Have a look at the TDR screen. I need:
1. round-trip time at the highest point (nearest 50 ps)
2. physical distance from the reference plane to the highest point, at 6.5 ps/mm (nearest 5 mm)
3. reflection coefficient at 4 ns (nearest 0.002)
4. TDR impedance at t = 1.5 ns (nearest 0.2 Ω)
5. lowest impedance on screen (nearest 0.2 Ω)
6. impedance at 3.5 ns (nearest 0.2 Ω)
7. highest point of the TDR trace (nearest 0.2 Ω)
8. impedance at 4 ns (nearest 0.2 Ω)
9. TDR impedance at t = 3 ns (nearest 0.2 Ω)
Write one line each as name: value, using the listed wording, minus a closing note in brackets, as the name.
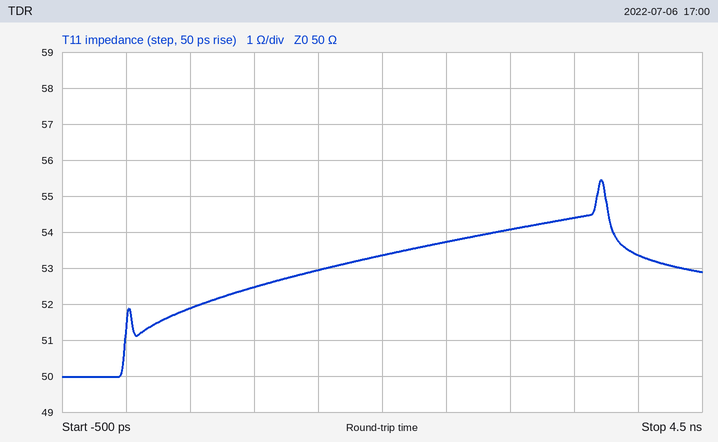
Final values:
round-trip time at the highest point: 3.70 ns
physical distance from the reference plane to the highest point, at 6.5 ps/mm: 285 mm
reflection coefficient at 4 ns: +0.032
TDR impedance at t = 1.5 ns: 53.0 Ω
lowest impedance on screen: 50.0 Ω
impedance at 3.5 ns: 54.4 Ω
highest point of the TDR trace: 55.4 Ω
impedance at 4 ns: 53.4 Ω
TDR impedance at t = 3 ns: 54.0 Ω
